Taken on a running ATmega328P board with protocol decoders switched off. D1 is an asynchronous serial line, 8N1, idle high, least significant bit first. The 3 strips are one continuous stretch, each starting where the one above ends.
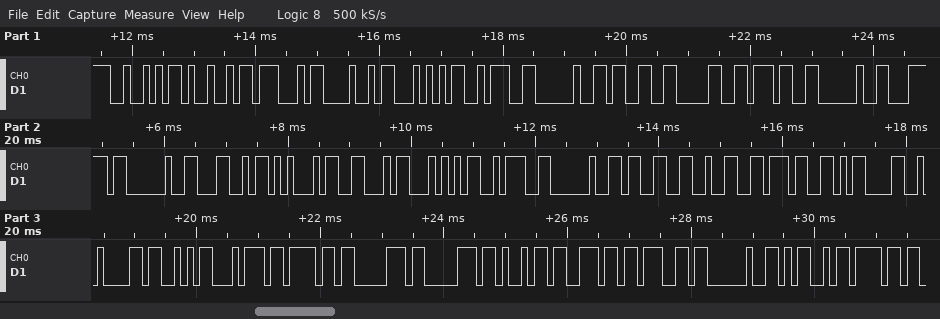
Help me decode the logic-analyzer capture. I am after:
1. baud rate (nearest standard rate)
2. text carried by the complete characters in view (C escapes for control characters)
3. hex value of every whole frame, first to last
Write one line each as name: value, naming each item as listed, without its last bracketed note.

baud rate: 9600 baud
text carried by the complete characters in view: "RIGHT: 307 | LEFT: 327\r\nStopping Mo"
hex value of every whole frame, first to last: 52 49 47 48 54 3A 20 33 30 37 20 7C 20 4C 45 46 54 3A 20 33 32 37 0D 0A 53 74 6F 70 70 69 6E 67 20 4D 6F
